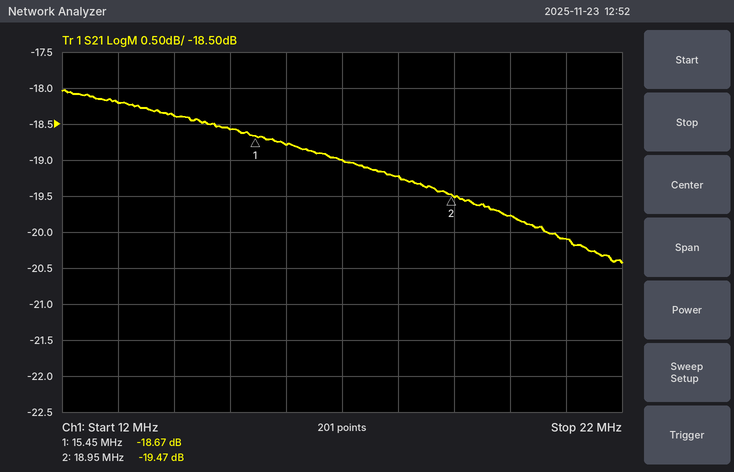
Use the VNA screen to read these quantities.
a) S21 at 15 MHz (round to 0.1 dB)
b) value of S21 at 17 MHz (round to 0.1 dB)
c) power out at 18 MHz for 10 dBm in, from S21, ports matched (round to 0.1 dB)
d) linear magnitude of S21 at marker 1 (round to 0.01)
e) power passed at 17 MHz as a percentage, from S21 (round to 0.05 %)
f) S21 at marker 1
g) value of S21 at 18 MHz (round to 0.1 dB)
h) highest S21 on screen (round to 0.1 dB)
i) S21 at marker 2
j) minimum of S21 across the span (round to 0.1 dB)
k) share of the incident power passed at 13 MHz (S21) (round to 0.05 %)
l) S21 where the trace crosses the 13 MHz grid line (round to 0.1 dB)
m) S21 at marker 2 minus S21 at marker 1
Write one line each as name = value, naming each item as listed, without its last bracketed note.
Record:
S21 at 15 MHz = -18.6 dB
value of S21 at 17 MHz = -19.0 dB
power out at 18 MHz for 10 dBm in, from S21, ports matched = -9.2 dBm
linear magnitude of S21 at marker 1 = 0.12
power passed at 17 MHz as a percentage, from S21 = 1.25 %
S21 at marker 1 = -18.67 dB
value of S21 at 18 MHz = -19.2 dB
highest S21 on screen = -18.0 dB
S21 at marker 2 = -19.47 dB
minimum of S21 across the span = -20.4 dB
share of the incident power passed at 13 MHz (S21) = 1.50 %
S21 where the trace crosses the 13 MHz grid line = -18.2 dB
S21 at marker 2 minus S21 at marker 1 = -0.80 dB
